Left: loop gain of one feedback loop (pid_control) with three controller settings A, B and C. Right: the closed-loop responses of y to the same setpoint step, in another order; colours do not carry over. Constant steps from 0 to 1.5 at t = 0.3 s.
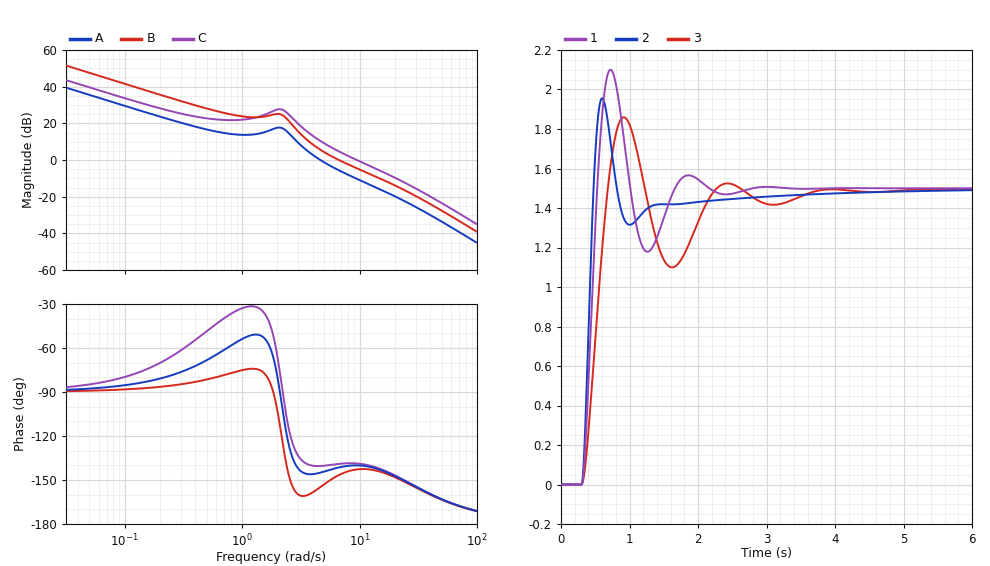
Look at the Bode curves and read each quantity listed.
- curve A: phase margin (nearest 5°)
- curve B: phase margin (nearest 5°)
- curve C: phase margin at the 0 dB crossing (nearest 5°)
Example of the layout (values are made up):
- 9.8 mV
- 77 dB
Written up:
- 35°
- 35°
- 40°
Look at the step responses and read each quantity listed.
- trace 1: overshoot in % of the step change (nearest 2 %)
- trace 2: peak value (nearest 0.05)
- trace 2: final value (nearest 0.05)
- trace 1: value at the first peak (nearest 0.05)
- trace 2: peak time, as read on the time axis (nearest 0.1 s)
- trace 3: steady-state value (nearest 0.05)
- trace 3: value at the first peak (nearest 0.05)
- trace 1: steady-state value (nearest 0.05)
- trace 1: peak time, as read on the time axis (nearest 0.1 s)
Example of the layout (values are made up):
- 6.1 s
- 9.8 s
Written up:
- 40 %
- 1.95
- 1.50
- 2.10
- 0.6 s
- 1.50
- 1.85
- 1.50
- 0.7 s
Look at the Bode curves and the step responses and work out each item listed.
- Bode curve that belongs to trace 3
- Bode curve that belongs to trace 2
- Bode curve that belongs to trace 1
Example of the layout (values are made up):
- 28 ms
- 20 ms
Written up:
- A
- C
- B
